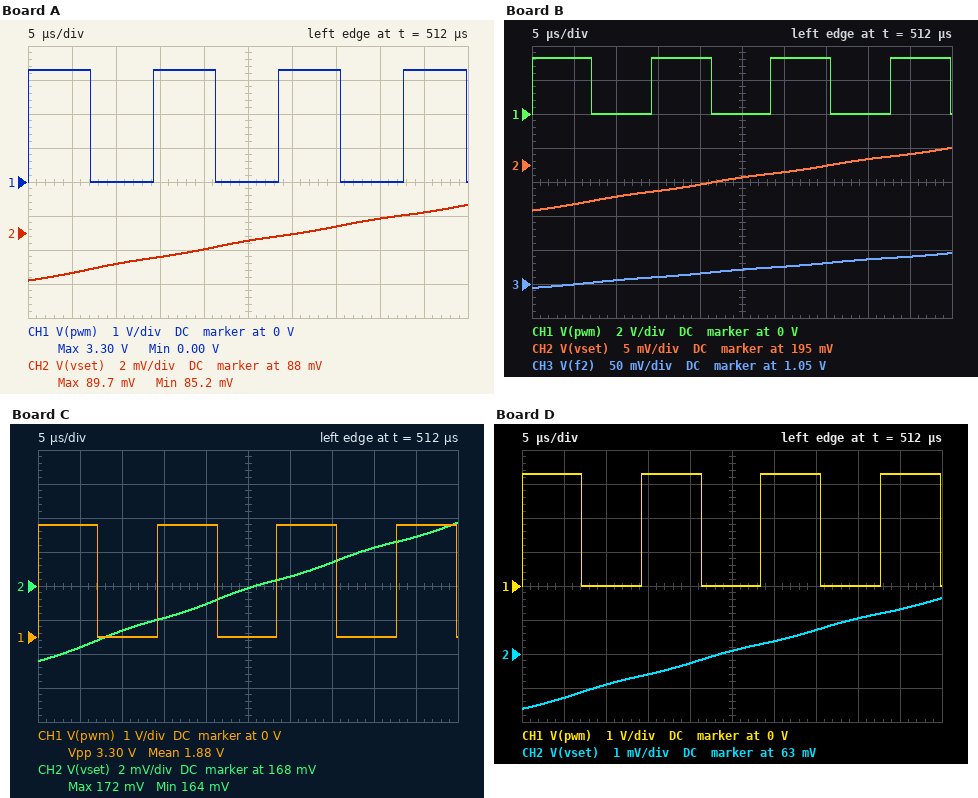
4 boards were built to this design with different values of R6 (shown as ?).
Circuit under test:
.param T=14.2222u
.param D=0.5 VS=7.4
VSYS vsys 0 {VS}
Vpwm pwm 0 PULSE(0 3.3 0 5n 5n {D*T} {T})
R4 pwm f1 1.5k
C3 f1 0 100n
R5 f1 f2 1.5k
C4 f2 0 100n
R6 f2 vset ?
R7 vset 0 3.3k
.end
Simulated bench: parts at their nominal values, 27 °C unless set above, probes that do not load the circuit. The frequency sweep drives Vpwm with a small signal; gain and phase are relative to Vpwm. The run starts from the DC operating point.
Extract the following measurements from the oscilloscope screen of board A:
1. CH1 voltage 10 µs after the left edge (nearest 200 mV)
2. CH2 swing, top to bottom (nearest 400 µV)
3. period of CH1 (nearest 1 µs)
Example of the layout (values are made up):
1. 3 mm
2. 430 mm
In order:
1. 0 V
2. 4.4 mV
3. 14 µs
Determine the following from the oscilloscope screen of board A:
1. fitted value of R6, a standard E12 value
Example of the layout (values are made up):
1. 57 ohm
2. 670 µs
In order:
1. 39 kΩ
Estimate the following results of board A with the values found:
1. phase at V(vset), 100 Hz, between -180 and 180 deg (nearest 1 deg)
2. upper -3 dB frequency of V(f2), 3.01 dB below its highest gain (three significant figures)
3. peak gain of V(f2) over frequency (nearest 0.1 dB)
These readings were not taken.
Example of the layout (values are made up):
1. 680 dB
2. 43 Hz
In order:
1. -15 deg
2. 423 Hz
3. -0.6 dB
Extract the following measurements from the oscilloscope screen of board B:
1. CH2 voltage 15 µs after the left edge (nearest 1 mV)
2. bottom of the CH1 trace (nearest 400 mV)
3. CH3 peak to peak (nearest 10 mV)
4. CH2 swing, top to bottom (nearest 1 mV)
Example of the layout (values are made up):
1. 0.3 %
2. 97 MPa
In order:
1. 191 mV
2. 0 V
3. 50 mV
4. 9 mV
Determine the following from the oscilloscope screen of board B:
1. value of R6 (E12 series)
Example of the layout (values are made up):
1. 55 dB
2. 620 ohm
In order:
1. 15 kΩ
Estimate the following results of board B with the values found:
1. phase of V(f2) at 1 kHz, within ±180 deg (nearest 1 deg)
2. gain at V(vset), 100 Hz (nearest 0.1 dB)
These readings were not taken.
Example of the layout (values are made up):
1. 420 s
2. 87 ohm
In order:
1. -85 deg
2. -16.4 dB
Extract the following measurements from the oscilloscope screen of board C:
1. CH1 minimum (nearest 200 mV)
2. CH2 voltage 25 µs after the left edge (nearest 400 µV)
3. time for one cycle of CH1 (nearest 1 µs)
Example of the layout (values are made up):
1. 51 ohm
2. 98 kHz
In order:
1. 0 V
2. 168.0 mV
3. 14 µs
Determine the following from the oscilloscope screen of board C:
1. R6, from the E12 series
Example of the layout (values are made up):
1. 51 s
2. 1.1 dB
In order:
1. 18 kΩ
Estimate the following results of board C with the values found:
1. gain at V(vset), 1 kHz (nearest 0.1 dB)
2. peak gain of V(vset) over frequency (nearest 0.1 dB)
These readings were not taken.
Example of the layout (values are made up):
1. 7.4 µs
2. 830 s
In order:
1. -25.5 dB
2. -17.3 dB
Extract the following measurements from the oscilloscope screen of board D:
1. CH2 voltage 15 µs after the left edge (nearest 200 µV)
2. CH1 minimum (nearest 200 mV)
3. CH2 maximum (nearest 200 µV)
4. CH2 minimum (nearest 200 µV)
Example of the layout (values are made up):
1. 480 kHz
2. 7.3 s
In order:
1. 62.4 mV
2. 0 V
3. 64.6 mV
4. 61.4 mV
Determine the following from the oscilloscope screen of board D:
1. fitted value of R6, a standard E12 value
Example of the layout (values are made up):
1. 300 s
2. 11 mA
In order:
1. 56 kΩ
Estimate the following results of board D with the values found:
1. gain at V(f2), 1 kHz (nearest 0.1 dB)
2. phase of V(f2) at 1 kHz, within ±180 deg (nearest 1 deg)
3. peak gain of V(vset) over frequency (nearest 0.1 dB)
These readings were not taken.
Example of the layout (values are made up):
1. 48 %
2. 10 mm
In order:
1. -9.1 dB
2. -87 deg
3. -25.5 dB
